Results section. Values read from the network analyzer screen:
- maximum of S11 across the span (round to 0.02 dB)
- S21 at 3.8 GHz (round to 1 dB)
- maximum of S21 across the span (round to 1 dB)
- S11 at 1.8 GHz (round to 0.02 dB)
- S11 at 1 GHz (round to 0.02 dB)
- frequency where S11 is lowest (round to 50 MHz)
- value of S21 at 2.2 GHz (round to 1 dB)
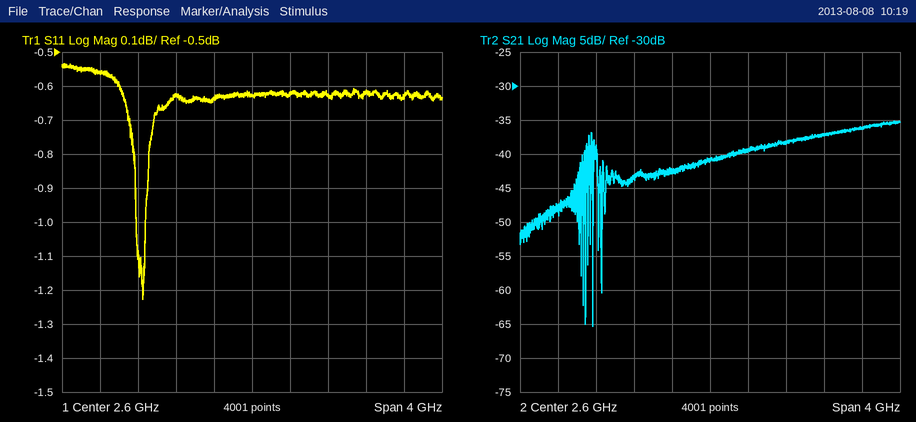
-0.54 dB
-37 dB
-35 dB
-0.62 dB
-0.56 dB
1.45 GHz
-42 dB
